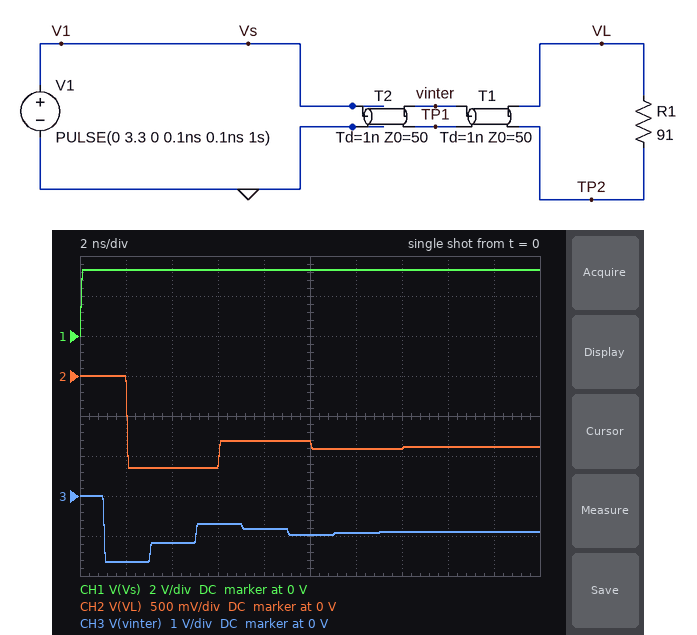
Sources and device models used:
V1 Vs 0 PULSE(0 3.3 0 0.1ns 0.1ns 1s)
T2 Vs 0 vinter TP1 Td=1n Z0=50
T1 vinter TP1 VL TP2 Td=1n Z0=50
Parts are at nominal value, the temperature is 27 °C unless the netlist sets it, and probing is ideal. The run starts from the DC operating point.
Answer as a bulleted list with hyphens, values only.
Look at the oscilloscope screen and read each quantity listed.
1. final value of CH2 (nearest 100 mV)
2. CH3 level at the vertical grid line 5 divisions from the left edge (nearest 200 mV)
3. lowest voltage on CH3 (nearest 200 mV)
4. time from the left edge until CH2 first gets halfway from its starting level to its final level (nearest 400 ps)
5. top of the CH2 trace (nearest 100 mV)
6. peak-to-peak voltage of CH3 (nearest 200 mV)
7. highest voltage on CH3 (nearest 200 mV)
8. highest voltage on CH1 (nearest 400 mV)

- -900 mV
- -1.0 V
- -1.6 V
- 2.0 ns
- 0 V
- 1.6 V
- 0 V
- 3.2 V
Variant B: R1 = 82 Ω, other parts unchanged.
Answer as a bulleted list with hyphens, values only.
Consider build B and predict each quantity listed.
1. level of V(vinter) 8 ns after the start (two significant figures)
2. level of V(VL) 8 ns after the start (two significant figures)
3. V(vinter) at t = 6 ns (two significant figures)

- -950 mV
- -930 mV
- -850 mV
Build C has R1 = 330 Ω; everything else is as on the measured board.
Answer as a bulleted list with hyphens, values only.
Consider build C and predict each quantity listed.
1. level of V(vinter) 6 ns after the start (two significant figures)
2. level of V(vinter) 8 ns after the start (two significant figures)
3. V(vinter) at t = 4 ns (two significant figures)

- 780 mV
- -110 mV
- -430 mV
